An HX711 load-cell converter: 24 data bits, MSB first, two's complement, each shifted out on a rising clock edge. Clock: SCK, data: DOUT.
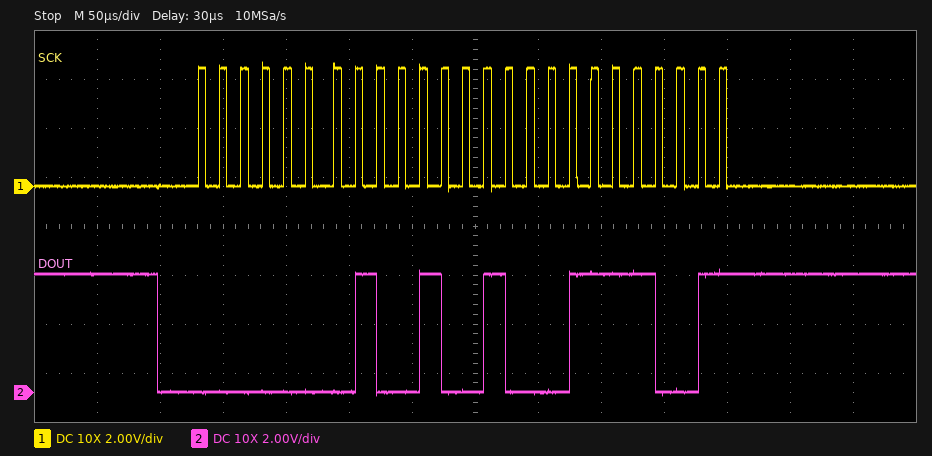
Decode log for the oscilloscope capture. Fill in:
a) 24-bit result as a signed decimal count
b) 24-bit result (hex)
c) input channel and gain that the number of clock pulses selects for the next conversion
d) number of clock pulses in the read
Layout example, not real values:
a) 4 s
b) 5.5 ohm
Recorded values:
a) 74873
b) 0x012479
c) channel A, gain 128
d) 25
